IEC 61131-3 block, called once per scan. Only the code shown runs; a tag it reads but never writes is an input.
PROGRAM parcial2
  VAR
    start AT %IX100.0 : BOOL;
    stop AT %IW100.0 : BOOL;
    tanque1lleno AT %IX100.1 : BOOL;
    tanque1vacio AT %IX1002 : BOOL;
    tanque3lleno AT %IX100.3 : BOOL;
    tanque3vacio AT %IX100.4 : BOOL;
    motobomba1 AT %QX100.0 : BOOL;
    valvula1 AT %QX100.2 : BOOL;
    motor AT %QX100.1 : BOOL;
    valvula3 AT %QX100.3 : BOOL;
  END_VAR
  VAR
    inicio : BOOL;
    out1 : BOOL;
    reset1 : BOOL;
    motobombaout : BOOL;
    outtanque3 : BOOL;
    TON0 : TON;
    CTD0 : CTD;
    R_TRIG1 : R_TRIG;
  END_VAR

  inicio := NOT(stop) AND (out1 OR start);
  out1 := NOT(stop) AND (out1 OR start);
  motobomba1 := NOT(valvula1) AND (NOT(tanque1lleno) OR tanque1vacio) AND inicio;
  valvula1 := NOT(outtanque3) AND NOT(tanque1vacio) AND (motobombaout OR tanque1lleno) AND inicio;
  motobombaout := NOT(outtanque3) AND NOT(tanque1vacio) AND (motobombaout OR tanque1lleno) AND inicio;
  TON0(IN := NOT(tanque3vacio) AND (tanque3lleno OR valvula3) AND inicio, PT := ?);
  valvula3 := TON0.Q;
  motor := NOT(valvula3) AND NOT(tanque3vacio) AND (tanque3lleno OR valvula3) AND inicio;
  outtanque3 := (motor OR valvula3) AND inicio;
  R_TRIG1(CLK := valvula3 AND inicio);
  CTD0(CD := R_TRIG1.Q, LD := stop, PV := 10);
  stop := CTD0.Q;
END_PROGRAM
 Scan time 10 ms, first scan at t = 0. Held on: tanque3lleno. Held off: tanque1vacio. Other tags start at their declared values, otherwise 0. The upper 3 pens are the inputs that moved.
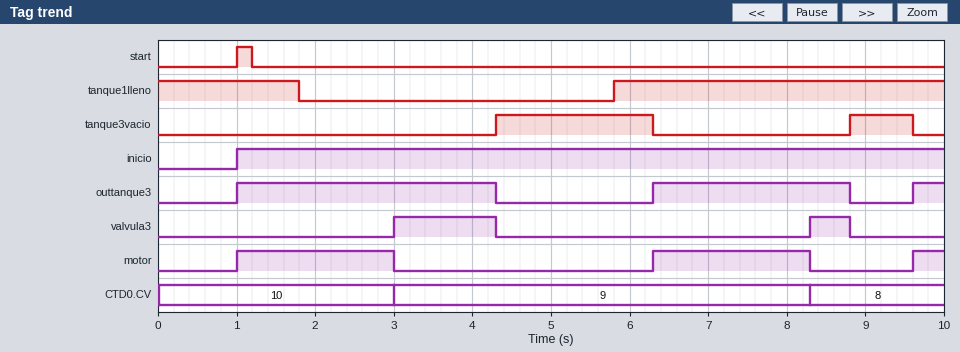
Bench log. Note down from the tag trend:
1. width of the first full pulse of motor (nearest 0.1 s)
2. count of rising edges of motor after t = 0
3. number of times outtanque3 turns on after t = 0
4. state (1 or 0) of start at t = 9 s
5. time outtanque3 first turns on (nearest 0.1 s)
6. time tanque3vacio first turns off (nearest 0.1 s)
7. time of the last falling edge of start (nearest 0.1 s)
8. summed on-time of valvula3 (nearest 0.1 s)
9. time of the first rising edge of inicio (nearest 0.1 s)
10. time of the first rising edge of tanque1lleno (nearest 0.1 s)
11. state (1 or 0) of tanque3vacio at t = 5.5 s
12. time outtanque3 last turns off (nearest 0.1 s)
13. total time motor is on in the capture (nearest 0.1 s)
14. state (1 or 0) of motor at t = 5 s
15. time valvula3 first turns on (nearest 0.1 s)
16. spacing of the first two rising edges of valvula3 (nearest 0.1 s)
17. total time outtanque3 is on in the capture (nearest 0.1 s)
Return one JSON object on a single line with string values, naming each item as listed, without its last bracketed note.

{"width of the first full pulse of motor": "2.0 s", "count of rising edges of motor after t = 0": "3", "number of times outtanque3 turns on after t = 0": "3", "state (1 or 0) of start at t = 9 s": "0", "time outtanque3 first turns on": "1.0 s", "time tanque3vacio first turns off": "6.3 s", "time of the last falling edge of start": "1.2 s", "summed on-time of valvula3": "1.8 s", "time of the first rising edge of inicio": "1.0 s", "time of the first rising edge of tanque1lleno": "5.8 s", "state (1 or 0) of tanque3vacio at t = 5.5 s": "1", "time outtanque3 last turns off": "8.8 s", "total time motor is on in the capture": "4.4 s", "state (1 or 0) of motor at t = 5 s": "0", "time valvula3 first turns on": "3.0 s", "spacing of the first two rising edges of valvula3": "5.3 s", "total time outtanque3 is on in the capture": "6.2 s"}
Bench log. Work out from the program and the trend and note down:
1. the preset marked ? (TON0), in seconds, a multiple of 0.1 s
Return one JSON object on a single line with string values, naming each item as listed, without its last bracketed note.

{"the preset marked ? (TON0), in seconds, a multiple of 0.1 s": "2.0 s"}
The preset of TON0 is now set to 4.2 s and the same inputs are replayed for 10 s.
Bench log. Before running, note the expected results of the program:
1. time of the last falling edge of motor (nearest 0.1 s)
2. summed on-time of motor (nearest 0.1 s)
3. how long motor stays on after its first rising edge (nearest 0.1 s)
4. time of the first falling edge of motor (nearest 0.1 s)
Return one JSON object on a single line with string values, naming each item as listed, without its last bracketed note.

{"time of the last falling edge of motor": "8.8 s", "summed on-time of motor": "6.2 s", "how long motor stays on after its first rising edge": "3.3 s", "time of the first falling edge of motor": "4.3 s"}
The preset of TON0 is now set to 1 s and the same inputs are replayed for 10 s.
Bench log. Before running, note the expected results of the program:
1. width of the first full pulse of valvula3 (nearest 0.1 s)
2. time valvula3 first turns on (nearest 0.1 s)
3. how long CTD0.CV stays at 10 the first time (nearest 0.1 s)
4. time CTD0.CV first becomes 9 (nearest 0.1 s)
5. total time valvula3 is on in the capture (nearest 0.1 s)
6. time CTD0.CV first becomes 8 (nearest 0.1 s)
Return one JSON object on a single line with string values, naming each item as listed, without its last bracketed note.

{"width of the first full pulse of valvula3": "2.3 s", "time valvula3 first turns on": "2.0 s", "how long CTD0.CV stays at 10 the first time": "2.0 s", "time CTD0.CV first becomes 9": "2.0 s", "total time valvula3 is on in the capture": "3.8 s", "time CTD0.CV first becomes 8": "7.3 s"}
